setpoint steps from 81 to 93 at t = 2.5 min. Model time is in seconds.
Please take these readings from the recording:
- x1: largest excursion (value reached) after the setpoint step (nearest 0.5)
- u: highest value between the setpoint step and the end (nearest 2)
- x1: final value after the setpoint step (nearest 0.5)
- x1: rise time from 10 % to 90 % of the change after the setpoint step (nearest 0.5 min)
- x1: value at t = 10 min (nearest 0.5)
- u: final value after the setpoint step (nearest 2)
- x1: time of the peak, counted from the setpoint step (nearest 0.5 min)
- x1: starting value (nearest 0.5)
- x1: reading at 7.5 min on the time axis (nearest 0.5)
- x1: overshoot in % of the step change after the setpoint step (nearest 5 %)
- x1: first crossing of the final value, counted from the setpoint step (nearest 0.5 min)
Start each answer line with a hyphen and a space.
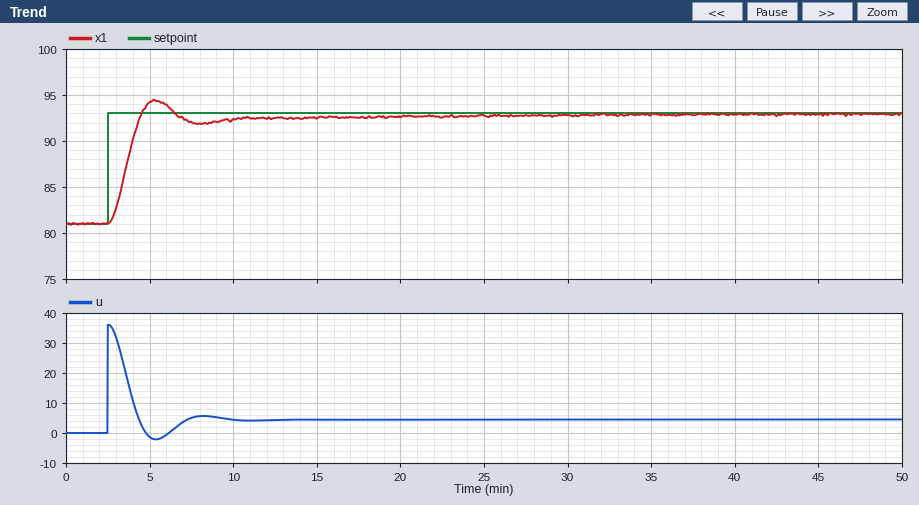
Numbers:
- 94.5
- 36
- 93.0
- 1.5 min
- 92.5
- 4
- 3.0 min
- 81.0
- 92.0
- 10 %
- 2.0 min
